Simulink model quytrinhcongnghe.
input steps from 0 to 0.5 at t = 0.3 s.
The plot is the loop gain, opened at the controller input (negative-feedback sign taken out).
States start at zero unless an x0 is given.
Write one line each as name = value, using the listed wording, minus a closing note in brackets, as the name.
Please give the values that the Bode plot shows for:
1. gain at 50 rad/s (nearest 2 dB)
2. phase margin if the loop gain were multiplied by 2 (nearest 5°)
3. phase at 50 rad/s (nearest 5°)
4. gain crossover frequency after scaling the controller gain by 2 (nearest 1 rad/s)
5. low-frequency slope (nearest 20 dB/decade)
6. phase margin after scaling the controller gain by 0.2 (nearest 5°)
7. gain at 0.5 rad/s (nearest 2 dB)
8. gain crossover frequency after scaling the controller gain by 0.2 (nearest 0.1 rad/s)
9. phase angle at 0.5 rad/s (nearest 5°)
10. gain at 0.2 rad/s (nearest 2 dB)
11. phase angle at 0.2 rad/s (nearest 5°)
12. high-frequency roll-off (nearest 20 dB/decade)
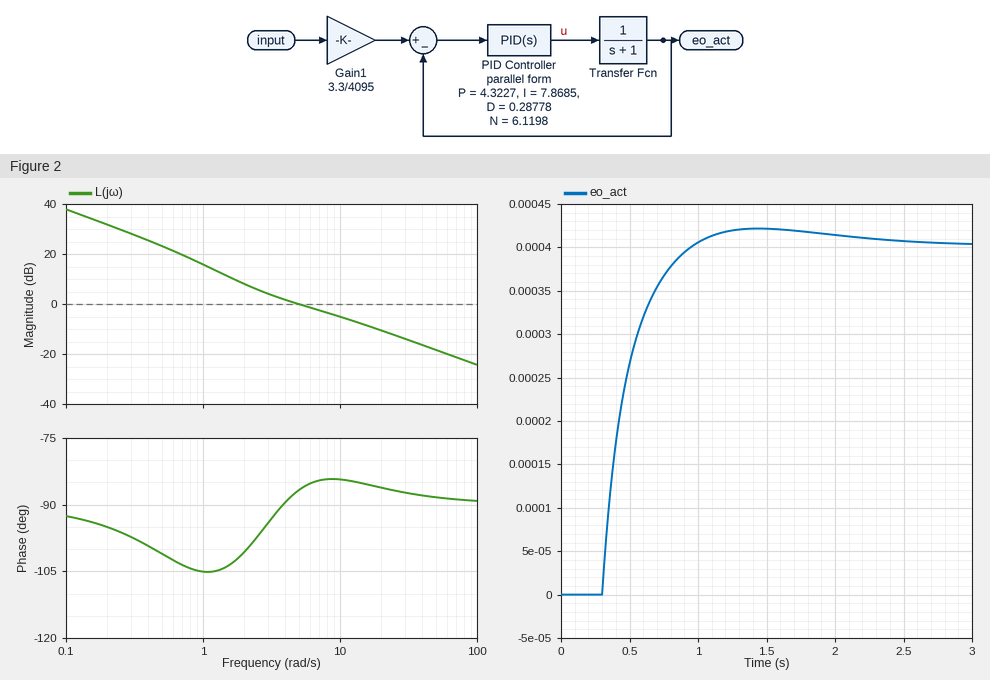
gain at 50 rad/s = -18 dB
phase margin if the loop gain were multiplied by 2 = 95°
phase at 50 rad/s = -90°
gain crossover frequency after scaling the controller gain by 2 = 11 rad/s
low-frequency slope = -20 dB/decade
phase margin after scaling the controller gain by 0.2 = 75°
gain at 0.5 rad/s = 24 dB
gain crossover frequency after scaling the controller gain by 0.2 = 1.2 rad/s
phase angle at 0.5 rad/s = -100°
gain at 0.2 rad/s = 32 dB
phase angle at 0.2 rad/s = -95°
high-frequency roll-off = -20 dB/decade
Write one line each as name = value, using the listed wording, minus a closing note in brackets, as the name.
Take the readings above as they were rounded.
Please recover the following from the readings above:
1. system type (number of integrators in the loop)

system type = 1
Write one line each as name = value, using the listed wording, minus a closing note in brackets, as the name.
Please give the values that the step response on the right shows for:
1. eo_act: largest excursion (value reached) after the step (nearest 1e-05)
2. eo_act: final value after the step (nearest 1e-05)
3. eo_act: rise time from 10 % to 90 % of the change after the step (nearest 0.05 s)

eo_act: largest excursion (value reached) after the step = 0.00042
eo_act: final value after the step = 0.00040
eo_act: rise time from 10 % to 90 % of the change after the step = 0.40 s
